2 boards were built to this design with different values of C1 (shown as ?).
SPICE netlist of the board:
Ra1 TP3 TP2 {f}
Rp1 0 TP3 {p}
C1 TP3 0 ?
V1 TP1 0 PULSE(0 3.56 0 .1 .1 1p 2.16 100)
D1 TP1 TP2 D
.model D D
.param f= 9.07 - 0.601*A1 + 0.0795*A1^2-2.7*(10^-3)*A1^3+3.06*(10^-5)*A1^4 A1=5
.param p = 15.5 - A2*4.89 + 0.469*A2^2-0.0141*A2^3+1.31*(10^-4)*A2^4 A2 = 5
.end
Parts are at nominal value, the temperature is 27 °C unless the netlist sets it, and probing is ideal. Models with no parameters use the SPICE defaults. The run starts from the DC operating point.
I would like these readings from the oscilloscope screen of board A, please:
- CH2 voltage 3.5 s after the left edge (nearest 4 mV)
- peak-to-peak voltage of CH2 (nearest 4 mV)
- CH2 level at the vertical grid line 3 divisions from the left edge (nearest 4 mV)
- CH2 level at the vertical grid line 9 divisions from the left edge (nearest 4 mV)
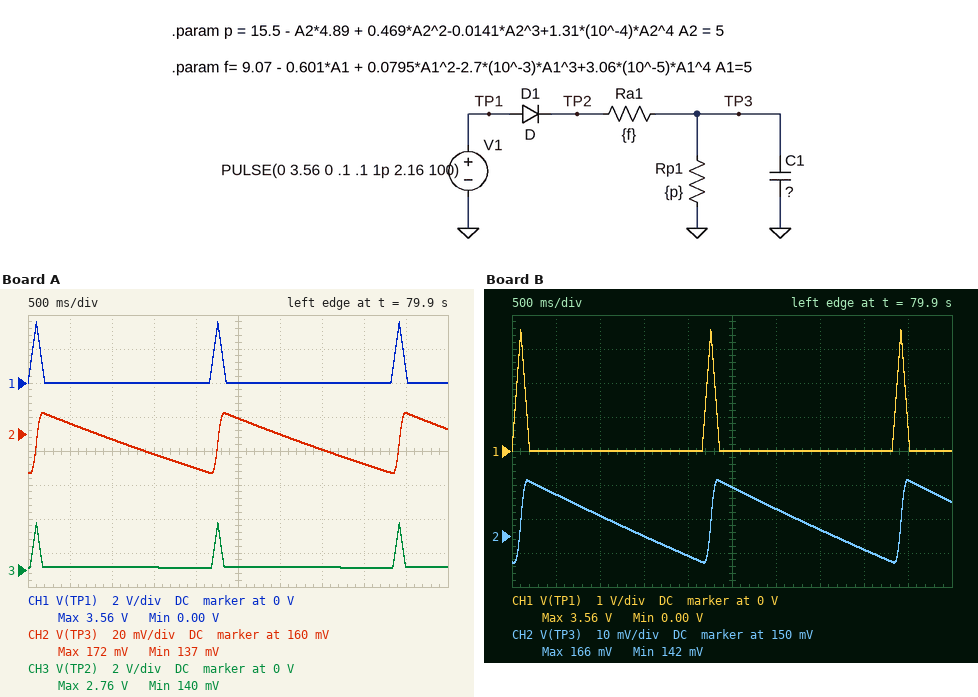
152 mV
36 mV
148 mV
172 mV
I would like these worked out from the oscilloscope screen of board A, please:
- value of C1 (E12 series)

560 mF
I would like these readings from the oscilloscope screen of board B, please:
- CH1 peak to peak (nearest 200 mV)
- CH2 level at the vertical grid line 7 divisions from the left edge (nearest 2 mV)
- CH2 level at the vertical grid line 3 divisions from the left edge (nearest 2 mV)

3.6 V
152 mV
150 mV
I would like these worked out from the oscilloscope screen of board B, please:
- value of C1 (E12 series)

820 mF
